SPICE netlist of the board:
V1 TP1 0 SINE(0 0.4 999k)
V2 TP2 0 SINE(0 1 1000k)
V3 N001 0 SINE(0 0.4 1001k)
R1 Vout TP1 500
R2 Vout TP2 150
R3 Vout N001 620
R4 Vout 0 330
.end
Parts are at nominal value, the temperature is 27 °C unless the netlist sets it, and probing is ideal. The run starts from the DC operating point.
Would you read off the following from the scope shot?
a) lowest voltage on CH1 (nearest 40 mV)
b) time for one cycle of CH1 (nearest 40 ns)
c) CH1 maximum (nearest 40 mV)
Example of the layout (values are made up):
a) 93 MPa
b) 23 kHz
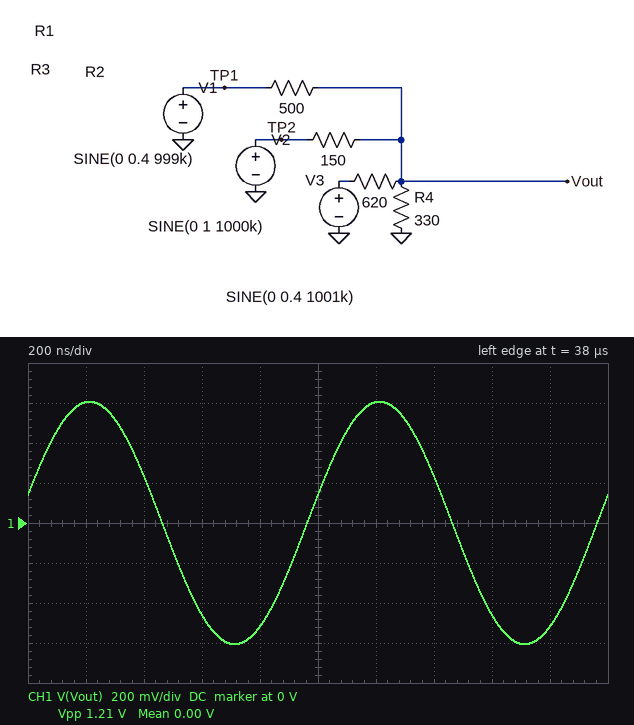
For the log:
a) -600 mV
b) 1.00 µs
c) 600 mV
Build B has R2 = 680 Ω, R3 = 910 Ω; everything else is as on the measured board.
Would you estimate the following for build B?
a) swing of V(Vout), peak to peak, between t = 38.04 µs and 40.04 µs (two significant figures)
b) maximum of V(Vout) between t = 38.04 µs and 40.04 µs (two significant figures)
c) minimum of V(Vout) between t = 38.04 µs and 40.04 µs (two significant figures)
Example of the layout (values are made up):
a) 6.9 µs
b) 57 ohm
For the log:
a) 700 mV
b) 350 mV
c) -350 mV
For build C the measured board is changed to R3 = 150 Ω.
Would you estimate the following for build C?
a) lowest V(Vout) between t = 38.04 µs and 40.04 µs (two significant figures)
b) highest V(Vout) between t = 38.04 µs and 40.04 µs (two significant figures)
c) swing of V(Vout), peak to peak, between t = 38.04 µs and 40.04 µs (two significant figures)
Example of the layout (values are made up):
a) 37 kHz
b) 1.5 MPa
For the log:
a) -550 mV
b) 550 mV
c) 1.1 V
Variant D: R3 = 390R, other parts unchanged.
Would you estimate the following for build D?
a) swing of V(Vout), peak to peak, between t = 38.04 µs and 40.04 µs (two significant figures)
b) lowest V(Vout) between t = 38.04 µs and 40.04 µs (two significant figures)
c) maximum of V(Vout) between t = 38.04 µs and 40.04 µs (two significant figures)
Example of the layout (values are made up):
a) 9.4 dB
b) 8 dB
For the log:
a) 1.2 V
b) -590 mV
c) 590 mV
